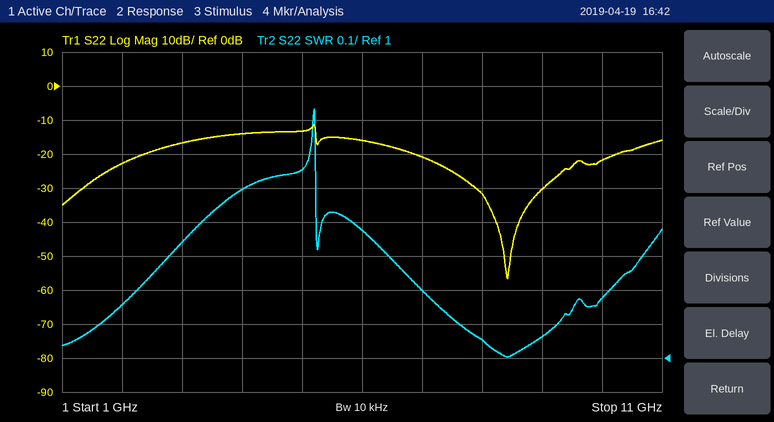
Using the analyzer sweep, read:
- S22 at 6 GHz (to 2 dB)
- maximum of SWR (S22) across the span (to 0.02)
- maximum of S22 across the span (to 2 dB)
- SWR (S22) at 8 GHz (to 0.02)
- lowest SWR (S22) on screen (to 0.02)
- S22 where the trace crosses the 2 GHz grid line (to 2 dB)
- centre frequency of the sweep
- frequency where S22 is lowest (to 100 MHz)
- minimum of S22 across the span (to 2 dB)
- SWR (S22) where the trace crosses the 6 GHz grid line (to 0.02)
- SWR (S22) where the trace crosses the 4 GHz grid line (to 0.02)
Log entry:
-16 dB
1.74
-12 dB
1.06
1.00
-22 dB
6 GHz
8.4 GHz
-56 dB
1.38
1.50
